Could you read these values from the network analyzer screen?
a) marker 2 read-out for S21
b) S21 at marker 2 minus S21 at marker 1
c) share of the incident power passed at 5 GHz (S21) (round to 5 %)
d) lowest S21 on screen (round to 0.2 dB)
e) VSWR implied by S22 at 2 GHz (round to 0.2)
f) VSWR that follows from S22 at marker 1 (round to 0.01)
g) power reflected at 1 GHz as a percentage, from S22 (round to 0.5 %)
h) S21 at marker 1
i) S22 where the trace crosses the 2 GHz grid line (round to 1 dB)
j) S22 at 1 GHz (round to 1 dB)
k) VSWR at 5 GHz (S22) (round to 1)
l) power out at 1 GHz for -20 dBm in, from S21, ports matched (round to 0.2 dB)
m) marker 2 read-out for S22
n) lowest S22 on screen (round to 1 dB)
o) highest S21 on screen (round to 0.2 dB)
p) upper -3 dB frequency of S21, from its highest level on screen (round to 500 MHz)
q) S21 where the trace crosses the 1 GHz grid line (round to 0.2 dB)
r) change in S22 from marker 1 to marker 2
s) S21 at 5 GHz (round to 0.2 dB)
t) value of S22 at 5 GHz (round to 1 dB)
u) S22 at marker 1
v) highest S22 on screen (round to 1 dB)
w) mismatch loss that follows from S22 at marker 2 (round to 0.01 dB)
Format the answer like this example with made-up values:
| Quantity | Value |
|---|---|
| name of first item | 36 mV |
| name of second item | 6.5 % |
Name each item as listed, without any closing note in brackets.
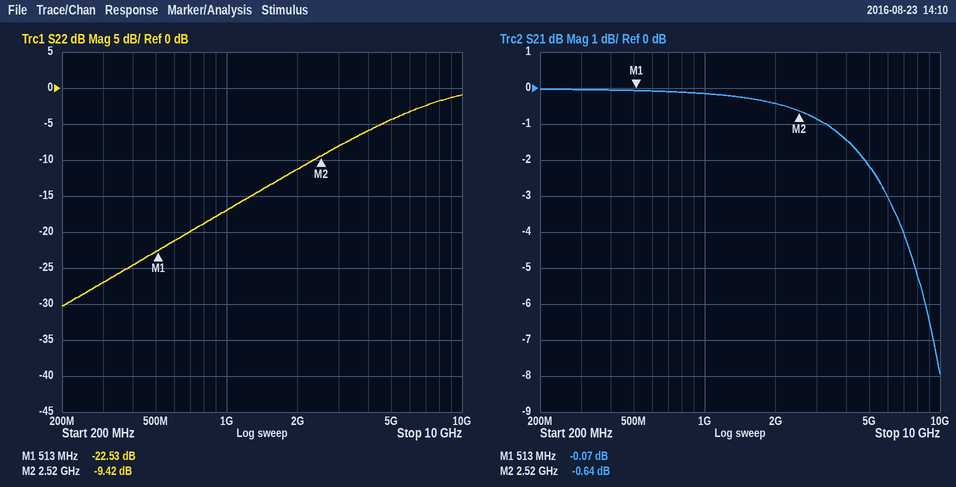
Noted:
| Quantity | Value |
|---|---|
| marker 2 read-out for S21 | -0.64 dB |
| S21 at marker 2 minus S21 at marker 1 | -0.57 dB |
| share of the incident power passed at 5 GHz (S21) | 60 % |
| lowest S21 on screen | -8.0 dB |
| VSWR implied by S22 at 2 GHz | 1.8 |
| VSWR that follows from S22 at marker 1 | 1.16 |
| power reflected at 1 GHz as a percentage, from S22 | 2.0 % |
| S21 at marker 1 | -0.07 dB |
| S22 where the trace crosses the 2 GHz grid line | -11 dB |
| S22 at 1 GHz | -17 dB |
| VSWR at 5 GHz (S22) | 4 |
| power out at 1 GHz for -20 dBm in, from S21, ports matched | -20.2 dBm |
| marker 2 read-out for S22 | -9.42 dB |
| lowest S22 on screen | -30 dB |
| highest S21 on screen | 0.0 dB |
| upper -3 dB frequency of S21, from its highest level on screen | 6.0 GHz |
| S21 where the trace crosses the 1 GHz grid line | -0.2 dB |
| change in S22 from marker 1 to marker 2 | 13.11 dB |
| S21 at 5 GHz | -2.2 dB |
| value of S22 at 5 GHz | -4 dB |
| S22 at marker 1 | -22.53 dB |
| highest S22 on screen | -1 dB |
| mismatch loss that follows from S22 at marker 2 | 0.53 dB |
